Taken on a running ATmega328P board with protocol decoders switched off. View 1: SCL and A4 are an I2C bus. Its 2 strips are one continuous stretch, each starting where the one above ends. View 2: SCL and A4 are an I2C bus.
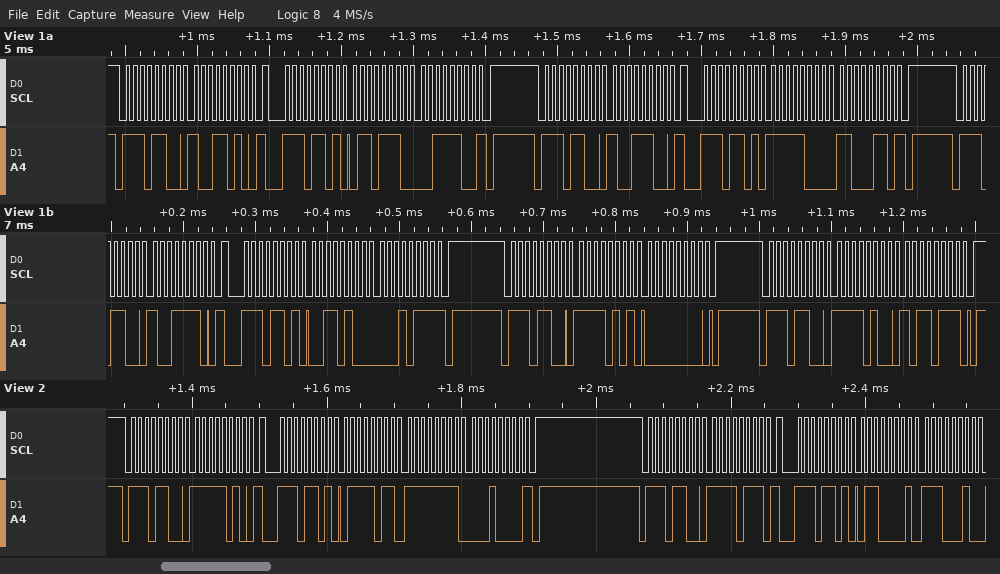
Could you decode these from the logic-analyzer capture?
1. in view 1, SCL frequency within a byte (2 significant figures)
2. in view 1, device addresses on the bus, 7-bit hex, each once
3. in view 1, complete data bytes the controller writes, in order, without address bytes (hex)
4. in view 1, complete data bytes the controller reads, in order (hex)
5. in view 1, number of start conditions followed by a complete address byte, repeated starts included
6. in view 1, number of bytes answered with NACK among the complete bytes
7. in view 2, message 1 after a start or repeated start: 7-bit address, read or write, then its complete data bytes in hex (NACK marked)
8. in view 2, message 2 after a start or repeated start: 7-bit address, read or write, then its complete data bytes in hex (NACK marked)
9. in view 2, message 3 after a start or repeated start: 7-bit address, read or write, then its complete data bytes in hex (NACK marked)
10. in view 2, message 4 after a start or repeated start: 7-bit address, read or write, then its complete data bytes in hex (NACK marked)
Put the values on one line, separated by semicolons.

100 kHz; 0x76; 9A 9C 9E F5 00 F4 B7; 6E 3C F8 C6 34 17; 8; 3; 0x76 write: FA; 0x76 read: 7B FF 10 NACK; 0x76 write: F7; 0x76 read: 61 E2
